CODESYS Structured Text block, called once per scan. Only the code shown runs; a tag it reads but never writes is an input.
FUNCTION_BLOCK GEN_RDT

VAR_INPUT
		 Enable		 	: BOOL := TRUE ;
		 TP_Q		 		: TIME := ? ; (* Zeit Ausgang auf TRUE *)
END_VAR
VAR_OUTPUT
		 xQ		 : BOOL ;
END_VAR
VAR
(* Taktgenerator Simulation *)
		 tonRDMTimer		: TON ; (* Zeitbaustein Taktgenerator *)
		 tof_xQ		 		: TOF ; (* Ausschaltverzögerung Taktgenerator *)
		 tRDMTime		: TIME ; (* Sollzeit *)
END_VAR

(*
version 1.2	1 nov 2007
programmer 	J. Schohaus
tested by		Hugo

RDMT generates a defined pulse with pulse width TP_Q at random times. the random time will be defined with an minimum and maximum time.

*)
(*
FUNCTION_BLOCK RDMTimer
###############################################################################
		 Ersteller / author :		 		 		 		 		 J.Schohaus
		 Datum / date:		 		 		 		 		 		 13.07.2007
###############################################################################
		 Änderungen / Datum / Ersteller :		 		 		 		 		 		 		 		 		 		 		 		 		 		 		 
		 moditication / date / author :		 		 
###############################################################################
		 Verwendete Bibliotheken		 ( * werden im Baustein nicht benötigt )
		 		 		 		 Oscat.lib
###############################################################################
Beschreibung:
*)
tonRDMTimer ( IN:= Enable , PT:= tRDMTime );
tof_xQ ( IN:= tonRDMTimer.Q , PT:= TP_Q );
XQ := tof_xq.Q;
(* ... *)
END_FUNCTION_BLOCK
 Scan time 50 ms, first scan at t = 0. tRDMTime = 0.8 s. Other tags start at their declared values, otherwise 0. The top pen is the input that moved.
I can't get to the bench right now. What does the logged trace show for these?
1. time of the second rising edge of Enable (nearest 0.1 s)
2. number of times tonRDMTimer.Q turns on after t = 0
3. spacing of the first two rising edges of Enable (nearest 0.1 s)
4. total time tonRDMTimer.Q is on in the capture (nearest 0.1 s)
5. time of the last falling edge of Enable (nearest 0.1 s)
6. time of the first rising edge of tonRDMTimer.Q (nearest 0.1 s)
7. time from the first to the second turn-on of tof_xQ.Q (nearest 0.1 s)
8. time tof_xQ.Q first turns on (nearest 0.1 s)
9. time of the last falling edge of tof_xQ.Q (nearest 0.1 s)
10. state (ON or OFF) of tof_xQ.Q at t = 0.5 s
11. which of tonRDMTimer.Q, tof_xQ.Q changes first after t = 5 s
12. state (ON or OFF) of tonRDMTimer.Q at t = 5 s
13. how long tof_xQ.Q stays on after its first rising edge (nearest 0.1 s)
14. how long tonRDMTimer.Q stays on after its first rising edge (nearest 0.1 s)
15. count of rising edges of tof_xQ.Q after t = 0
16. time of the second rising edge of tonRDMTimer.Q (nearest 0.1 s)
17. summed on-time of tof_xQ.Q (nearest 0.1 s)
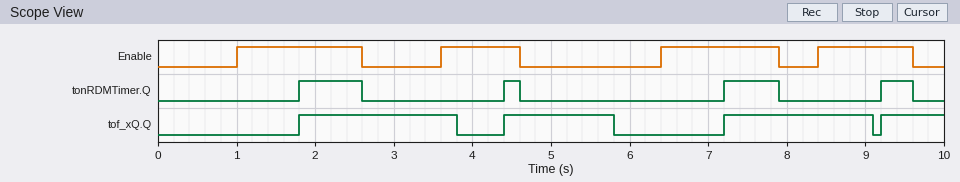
3.6 s
4
2.6 s
2.1 s
9.6 s
1.8 s
2.6 s
1.8 s
9.1 s
OFF
tof_xQ.Q
OFF
2.0 s
0.8 s
4
4.4 s
6.1 s
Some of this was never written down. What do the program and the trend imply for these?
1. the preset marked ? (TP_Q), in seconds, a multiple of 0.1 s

1.2 s
